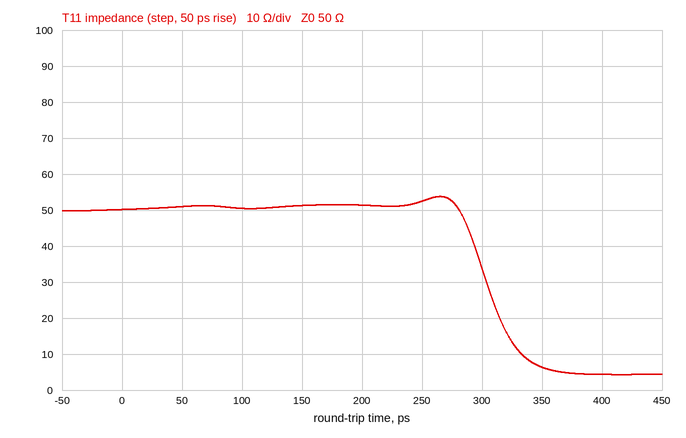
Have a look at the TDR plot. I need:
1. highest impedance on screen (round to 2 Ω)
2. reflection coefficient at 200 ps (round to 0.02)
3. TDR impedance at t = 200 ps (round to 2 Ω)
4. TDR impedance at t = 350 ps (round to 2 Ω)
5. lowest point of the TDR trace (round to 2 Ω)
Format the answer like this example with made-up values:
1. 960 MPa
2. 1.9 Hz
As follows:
1. 54 Ω
2. +0.02
3. 52 Ω
4. 6 Ω
5. 4 Ω
